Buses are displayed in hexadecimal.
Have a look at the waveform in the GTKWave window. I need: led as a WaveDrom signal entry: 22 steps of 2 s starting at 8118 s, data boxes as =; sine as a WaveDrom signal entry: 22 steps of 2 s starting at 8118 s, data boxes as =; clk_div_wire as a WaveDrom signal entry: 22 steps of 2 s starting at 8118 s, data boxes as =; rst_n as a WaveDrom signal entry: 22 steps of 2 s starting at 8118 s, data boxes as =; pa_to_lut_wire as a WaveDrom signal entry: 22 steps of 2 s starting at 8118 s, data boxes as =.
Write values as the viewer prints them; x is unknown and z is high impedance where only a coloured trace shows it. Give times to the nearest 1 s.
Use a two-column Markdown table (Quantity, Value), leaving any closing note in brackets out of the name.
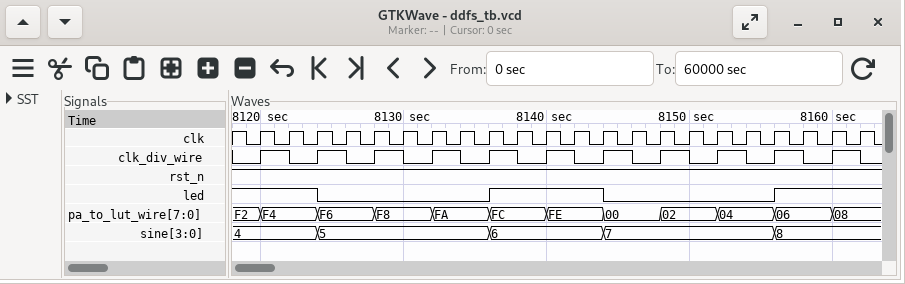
| Quantity | Value |
|---|---|
| led as a WaveDrom signal entry: 22 steps of 2 s starting at 8118 s, data boxes as = | {name: 'led', wave: '1..0.....1...0.....1..'} |
| sine as a WaveDrom signal entry: 22 steps of 2 s starting at 8118 s, data boxes as = | {name: 'sine', wave: '=..=.....=...=.....=..', data: '4 5 6 7 8'} |
| clk_div_wire as a WaveDrom signal entry: 22 steps of 2 s starting at 8118 s, data boxes as = | {name: 'clk_div_wire', wave: '0101010101010101010101'} |
| rst_n as a WaveDrom signal entry: 22 steps of 2 s starting at 8118 s, data boxes as = | {name: 'rst_n', wave: '1.....................'} |
| pa_to_lut_wire as a WaveDrom signal entry: 22 steps of 2 s starting at 8118 s, data boxes as = | {name: 'pa_to_lut_wire', wave: '==.=.=.=.=.=.=.=.=.=.=', data: 'F2 F4 F6 F8 FA FC FE 00 02 04 06 08'} |
